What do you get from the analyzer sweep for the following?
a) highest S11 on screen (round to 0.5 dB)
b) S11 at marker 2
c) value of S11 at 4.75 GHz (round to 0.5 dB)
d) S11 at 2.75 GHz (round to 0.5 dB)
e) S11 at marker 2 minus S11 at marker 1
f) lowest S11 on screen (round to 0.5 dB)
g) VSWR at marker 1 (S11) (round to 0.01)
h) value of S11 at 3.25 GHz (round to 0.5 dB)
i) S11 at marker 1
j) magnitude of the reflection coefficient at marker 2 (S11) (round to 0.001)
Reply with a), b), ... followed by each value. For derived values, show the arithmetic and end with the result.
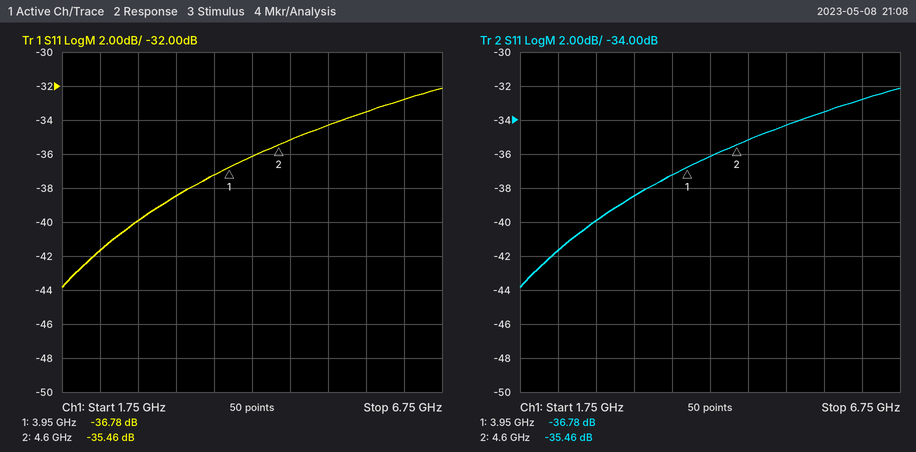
a) -32.0 dB
b) -35.46 dB
c) -35.0 dB
d) -40.0 dB
e) -35.46 − (-36.78) = 1.32 dB
f) -44.0 dB
g) (1 + 0.0145)/(1 − 0.0145) ≈ 1.03
h) -38.5 dB
i) -36.78 dB
j) 10^(-35.46/20) ≈ 0.017
